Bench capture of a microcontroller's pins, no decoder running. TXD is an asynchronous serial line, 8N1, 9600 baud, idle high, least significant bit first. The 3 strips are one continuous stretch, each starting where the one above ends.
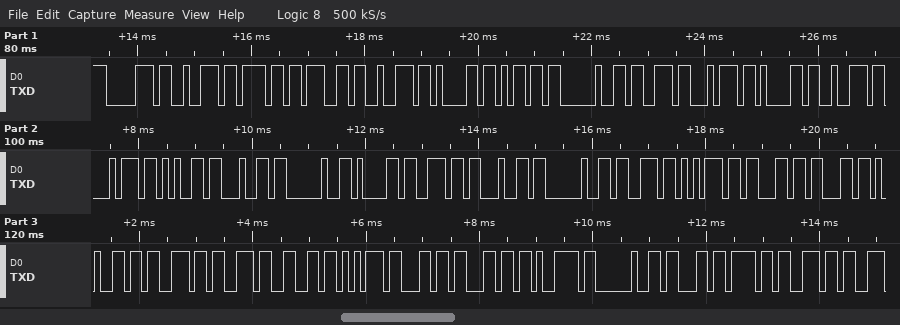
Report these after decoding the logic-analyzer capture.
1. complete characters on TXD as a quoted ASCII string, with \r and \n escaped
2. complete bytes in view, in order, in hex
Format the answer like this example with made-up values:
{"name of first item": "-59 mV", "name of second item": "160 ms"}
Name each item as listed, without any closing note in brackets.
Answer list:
{"complete characters on TXD as a quoted ASCII string, with \\r and \\n escaped": "\"program started and successfully con\"", "complete bytes in view, in order, in hex": "70 72 6F 67 72 61 6D 20 73 74 61 72 74 65 64 20 61 6E 64 20 73 75 63 63 65 73 73 66 75 6C 6C 79 20 63 6F 6E"}
